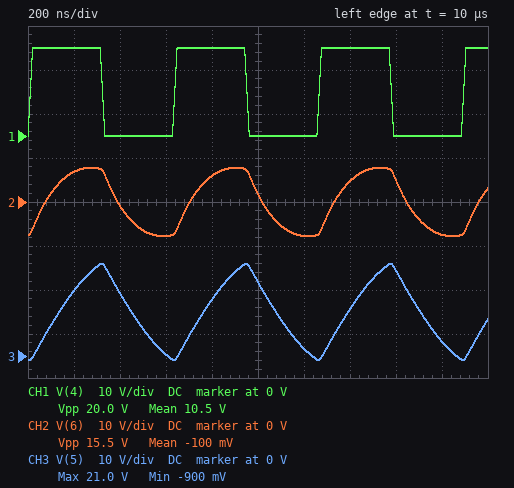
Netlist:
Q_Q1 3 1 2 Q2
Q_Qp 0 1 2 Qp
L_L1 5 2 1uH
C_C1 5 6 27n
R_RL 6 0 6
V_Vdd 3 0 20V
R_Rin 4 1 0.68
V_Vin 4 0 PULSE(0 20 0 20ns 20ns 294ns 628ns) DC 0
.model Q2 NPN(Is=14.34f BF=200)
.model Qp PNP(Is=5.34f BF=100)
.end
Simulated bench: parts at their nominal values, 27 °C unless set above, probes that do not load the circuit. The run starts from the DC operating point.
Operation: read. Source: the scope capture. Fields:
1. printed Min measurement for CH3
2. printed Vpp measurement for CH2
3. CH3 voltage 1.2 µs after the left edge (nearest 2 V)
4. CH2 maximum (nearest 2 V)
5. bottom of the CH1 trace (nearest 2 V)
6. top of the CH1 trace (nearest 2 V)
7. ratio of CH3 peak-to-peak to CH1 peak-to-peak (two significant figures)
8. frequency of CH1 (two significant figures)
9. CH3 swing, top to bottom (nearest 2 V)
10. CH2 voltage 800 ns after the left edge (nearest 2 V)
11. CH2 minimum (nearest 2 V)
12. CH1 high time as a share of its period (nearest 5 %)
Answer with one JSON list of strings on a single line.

["-900 mV", "15.5 V", "2 V", "8 V", "0 V", "20 V", "1.1", "1.6 MHz", "22 V", "6 V", "-8 V", "50 %"]
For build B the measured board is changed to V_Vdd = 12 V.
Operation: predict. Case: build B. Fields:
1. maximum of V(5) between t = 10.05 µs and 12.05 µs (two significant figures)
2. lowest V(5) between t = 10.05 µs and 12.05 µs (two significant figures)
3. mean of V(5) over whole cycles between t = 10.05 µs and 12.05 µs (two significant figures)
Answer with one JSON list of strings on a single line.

["13 V", "-220 mV", "6.4 V"]
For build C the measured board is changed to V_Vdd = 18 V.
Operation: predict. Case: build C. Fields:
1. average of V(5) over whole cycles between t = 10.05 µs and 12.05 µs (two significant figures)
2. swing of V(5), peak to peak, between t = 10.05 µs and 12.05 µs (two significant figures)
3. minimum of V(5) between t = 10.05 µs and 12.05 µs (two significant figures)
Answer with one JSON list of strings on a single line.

["9.3 V", "20 V", "-740 mV"]
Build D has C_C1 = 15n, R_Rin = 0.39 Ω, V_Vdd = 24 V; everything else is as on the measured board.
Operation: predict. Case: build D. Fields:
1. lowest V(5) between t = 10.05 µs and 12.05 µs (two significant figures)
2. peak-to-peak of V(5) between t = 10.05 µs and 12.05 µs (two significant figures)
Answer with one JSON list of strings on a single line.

["-6.5 V", "33 V"]
